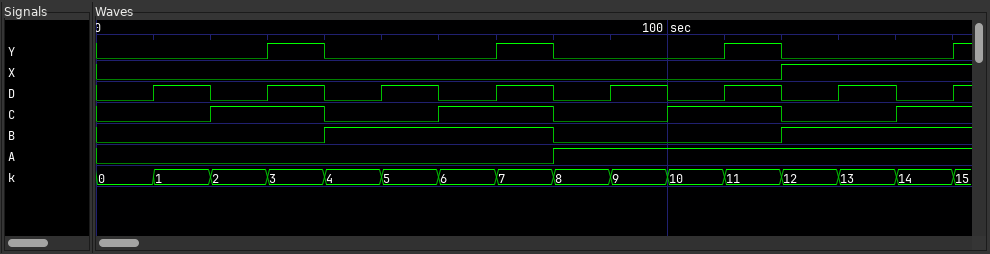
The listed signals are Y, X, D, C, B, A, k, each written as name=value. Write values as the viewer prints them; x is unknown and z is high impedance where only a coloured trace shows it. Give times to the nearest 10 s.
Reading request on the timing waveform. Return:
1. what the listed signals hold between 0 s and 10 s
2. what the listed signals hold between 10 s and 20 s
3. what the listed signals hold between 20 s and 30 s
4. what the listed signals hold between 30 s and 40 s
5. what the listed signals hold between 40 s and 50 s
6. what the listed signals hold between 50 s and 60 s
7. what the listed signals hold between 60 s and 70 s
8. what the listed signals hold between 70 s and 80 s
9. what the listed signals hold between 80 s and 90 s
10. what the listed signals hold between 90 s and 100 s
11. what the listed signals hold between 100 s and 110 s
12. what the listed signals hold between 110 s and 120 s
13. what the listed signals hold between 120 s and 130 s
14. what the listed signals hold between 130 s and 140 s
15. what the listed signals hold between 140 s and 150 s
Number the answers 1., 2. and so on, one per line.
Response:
1. Y=0, X=0, D=0, C=0, B=0, A=0, k=0
2. Y=0, X=0, D=1, C=0, B=0, A=0, k=1
3. Y=0, X=0, D=0, C=1, B=0, A=0, k=2
4. Y=1, X=0, D=1, C=1, B=0, A=0, k=3
5. Y=0, X=0, D=0, C=0, B=1, A=0, k=4
6. Y=0, X=0, D=1, C=0, B=1, A=0, k=5
7. Y=0, X=0, D=0, C=1, B=1, A=0, k=6
8. Y=1, X=0, D=1, C=1, B=1, A=0, k=7
9. Y=0, X=0, D=0, C=0, B=0, A=1, k=8
10. Y=0, X=0, D=1, C=0, B=0, A=1, k=9
11. Y=0, X=0, D=0, C=1, B=0, A=1, k=10
12. Y=1, X=0, D=1, C=1, B=0, A=1, k=11
13. Y=0, X=1, D=0, C=0, B=1, A=1, k=12
14. Y=0, X=1, D=1, C=0, B=1, A=1, k=13
15. Y=0, X=1, D=0, C=1, B=1, A=1, k=14
